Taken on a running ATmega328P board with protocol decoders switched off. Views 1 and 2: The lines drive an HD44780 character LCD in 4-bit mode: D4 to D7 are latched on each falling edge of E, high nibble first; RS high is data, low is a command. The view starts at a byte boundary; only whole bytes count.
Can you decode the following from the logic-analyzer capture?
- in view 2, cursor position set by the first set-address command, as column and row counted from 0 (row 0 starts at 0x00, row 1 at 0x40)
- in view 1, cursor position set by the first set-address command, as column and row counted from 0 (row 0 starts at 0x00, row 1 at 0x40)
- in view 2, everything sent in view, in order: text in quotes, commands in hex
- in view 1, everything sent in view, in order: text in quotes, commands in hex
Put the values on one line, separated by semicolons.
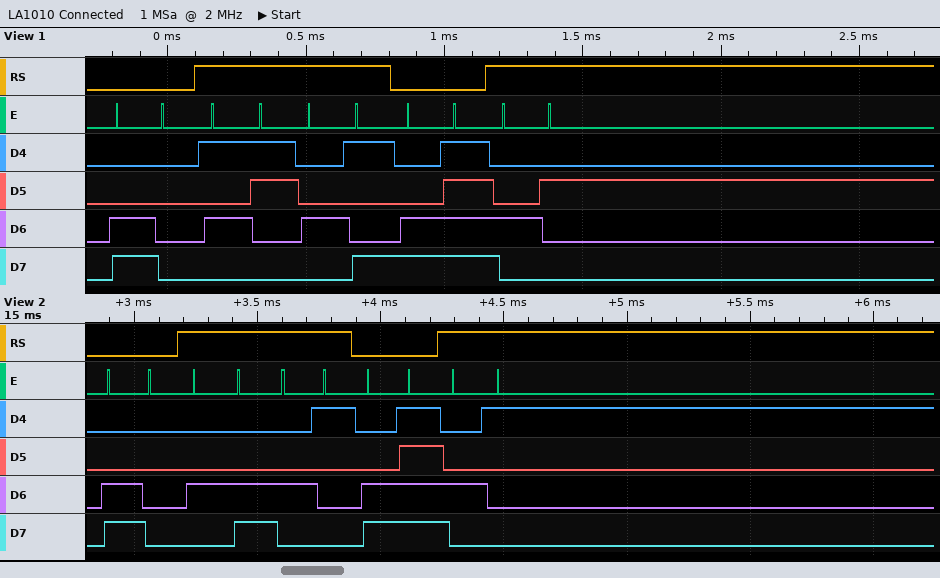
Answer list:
column 0, row 1; column 0, row 1; 0xC0 "LA" 0xCF "A"; 0xC0 "SI" 0xCF "B"
